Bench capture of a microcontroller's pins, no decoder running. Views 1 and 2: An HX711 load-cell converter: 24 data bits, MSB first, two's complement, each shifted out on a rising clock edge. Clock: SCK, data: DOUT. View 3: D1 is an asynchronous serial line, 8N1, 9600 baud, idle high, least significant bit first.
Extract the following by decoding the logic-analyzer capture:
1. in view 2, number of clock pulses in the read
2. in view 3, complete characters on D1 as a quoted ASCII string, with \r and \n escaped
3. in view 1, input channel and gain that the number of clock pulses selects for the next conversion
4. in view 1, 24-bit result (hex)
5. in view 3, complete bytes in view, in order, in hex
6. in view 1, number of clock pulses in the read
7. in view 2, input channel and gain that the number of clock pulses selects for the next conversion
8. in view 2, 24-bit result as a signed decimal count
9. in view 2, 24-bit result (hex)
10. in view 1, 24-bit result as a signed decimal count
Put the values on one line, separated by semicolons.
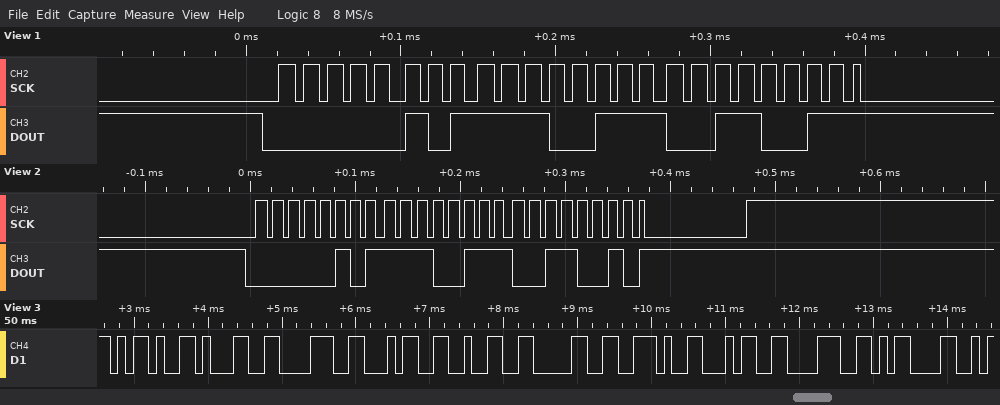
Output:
26; "-18420.48\r"; channel A, gain 128; 0x05E733; 2D 31 38 34 32 30 2E 34 38 0D; 25; channel B, gain 32; 386866; 0x05E732; 386867
